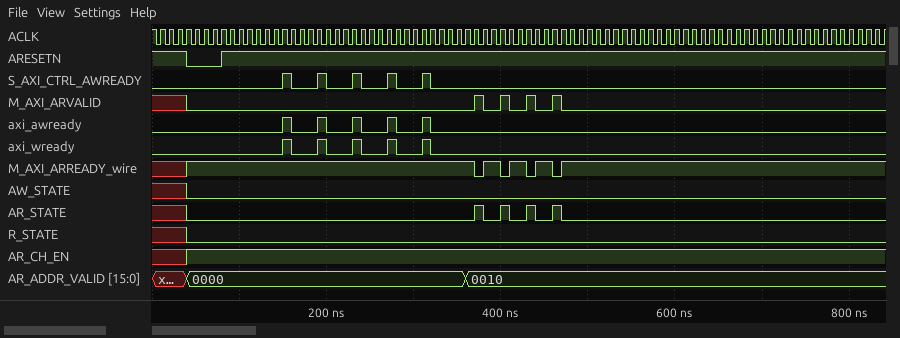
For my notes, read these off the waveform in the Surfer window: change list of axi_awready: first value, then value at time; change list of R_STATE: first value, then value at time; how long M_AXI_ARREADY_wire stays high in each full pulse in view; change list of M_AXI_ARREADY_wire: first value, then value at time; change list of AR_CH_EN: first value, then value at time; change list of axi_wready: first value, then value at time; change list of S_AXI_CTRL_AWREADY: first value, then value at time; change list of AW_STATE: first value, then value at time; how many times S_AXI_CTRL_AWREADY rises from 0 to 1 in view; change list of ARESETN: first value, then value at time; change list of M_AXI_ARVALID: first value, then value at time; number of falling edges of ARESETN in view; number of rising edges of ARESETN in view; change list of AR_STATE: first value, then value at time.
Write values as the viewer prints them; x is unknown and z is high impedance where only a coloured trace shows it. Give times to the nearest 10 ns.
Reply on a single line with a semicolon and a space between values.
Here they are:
0, 1 at 150 ns, 0 at 160 ns, 1 at 190 ns, 0 at 200 ns, 1 at 230 ns, 0 at 240 ns, 1 at 270 ns, 0 at 280 ns, 1 at 310 ns, 0 at 320 ns; x, 0 at 40 ns; 20 ns, 20 ns, 20 ns; x, 1 at 40 ns, 0 at 370 ns, 1 at 380 ns, 0 at 400 ns, 1 at 410 ns, 0 at 430 ns, 1 at 440 ns, 0 at 460 ns, 1 at 470 ns; x, 1 at 40 ns; 0, 1 at 150 ns, 0 at 160 ns, 1 at 190 ns, 0 at 200 ns, 1 at 230 ns, 0 at 240 ns, 1 at 270 ns, 0 at 280 ns, 1 at 310 ns, 0 at 320 ns; 0, 1 at 150 ns, 0 at 160 ns, 1 at 190 ns, 0 at 200 ns, 1 at 230 ns, 0 at 240 ns, 1 at 270 ns, 0 at 280 ns, 1 at 310 ns, 0 at 320 ns; x, 0 at 40 ns; 5; 1, 0 at 40 ns, 1 at 80 ns; x, 0 at 40 ns, 1 at 370 ns, 0 at 380 ns, 1 at 400 ns, 0 at 410 ns, 1 at 430 ns, 0 at 440 ns, 1 at 460 ns, 0 at 470 ns; 1; 1; x, 0 at 40 ns, 1 at 370 ns, 0 at 380 ns, 1 at 400 ns, 0 at 410 ns, 1 at 430 ns, 0 at 440 ns, 1 at 460 ns, 0 at 470 ns
